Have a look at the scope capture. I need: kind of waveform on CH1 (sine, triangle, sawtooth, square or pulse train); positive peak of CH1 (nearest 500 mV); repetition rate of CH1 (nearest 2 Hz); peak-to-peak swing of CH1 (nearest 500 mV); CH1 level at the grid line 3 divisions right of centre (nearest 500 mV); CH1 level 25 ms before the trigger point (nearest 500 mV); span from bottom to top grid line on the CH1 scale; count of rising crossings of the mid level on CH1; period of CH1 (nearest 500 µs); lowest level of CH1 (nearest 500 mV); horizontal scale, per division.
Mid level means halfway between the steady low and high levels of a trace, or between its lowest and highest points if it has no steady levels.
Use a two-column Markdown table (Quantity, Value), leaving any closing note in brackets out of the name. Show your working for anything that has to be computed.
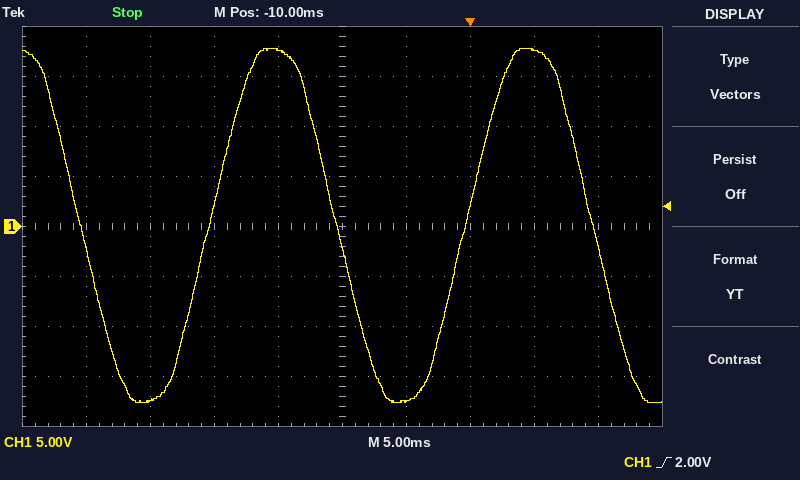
| Quantity | Value |
|---|---|
| kind of waveform on CH1 | sine |
| positive peak of CH1 | 18.0 V |
| repetition rate of CH1 | 1 / 20.0 ms ≈ 50 Hz |
| peak-to-peak swing of CH1 | 18.0 V − (-17.5 V) = 35.5 V |
| CH1 level at the grid line 3 divisions right of centre | 17.5 V |
| CH1 level 25 ms before the trigger point | -17.5 V |
| span from bottom to top grid line on the CH1 scale | 40 V |
| count of rising crossings of the mid level on CH1 | 2 |
| period of CH1 | 20.0 ms |
| lowest level of CH1 | -17.5 V |
| horizontal scale, per division | 5 ms |
